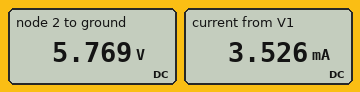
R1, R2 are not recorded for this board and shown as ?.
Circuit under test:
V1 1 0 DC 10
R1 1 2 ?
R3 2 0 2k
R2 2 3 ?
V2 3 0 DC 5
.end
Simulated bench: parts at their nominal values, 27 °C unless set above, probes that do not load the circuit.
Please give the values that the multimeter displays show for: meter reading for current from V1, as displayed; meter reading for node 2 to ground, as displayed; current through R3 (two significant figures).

3.526 mA
5.769 V
2.9 mA
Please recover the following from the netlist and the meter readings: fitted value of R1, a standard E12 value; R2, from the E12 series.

1.2 kΩ
1.2 kΩ
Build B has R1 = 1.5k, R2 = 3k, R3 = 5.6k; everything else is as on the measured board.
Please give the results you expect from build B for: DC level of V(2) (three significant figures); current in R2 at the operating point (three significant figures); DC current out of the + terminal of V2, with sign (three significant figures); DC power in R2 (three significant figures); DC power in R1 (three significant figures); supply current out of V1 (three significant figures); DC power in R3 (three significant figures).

7.07 V
690 µA
-690 µA
1.43 mW
5.72 mW
1.95 mA
8.93 mW
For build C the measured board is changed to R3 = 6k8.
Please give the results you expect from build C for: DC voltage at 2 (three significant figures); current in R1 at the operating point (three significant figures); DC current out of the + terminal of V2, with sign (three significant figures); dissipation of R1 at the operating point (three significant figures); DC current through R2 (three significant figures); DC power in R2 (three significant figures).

6.89 V
2.59 mA
-1.58 mA
8.05 mW
1.58 mA
2.98 mW
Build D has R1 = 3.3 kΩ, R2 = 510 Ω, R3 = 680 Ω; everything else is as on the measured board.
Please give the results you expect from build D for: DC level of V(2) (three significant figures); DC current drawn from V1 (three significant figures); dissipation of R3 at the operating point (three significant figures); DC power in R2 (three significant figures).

3.44 V
1.99 mA
17.4 mW
4.79 mW
